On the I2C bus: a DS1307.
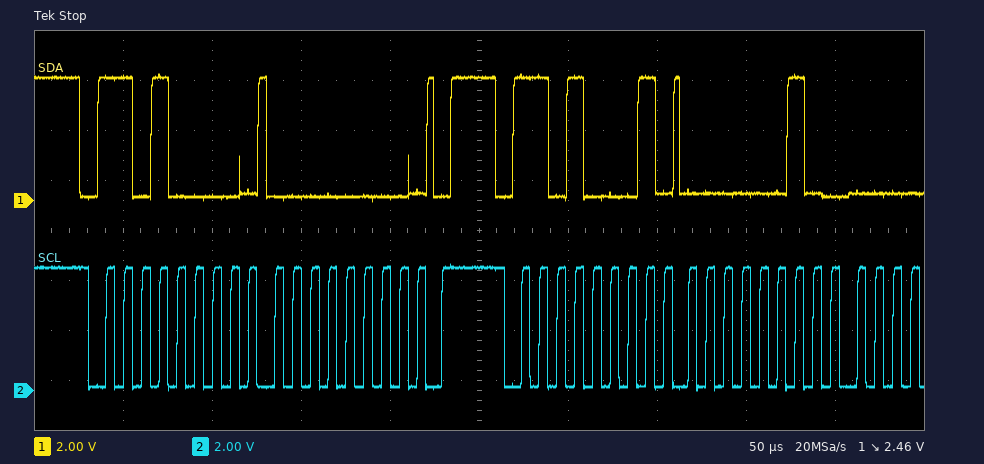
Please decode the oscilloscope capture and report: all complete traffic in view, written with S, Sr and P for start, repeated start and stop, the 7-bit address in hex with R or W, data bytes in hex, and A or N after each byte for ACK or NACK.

S 68W A 00 A P S 68R A 02 A
